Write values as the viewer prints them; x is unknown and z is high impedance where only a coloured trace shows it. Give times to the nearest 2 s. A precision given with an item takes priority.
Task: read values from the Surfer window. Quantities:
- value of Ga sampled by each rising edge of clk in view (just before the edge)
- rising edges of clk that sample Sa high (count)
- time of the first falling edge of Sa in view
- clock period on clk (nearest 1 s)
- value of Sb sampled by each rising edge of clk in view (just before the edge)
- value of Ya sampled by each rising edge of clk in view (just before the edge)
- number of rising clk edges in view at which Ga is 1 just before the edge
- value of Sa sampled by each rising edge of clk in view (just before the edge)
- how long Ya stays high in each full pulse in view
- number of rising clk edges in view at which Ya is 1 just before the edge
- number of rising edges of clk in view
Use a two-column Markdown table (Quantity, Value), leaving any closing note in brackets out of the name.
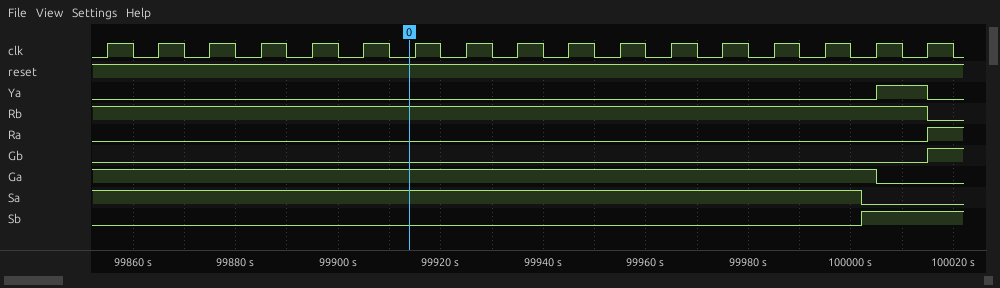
| Quantity | Value |
|---|---|
| value of Ga sampled by each rising edge of clk in view | 1 1 1 1 1 1 1 1 1 1 1 1 1 1 1 1 0 |
| rising edges of clk that sample Sa high | 15 |
| time of the first falling edge of Sa in view | 100002 s |
| clock period on clk | 10 s |
| value of Sb sampled by each rising edge of clk in view | 0 0 0 0 0 0 0 0 0 0 0 0 0 0 0 1 1 |
| value of Ya sampled by each rising edge of clk in view | 0 0 0 0 0 0 0 0 0 0 0 0 0 0 0 0 1 |
| number of rising clk edges in view at which Ga is 1 just before the edge | 16 |
| value of Sa sampled by each rising edge of clk in view | 1 1 1 1 1 1 1 1 1 1 1 1 1 1 1 0 0 |
| how long Ya stays high in each full pulse in view | 10 s |
| number of rising clk edges in view at which Ya is 1 just before the edge | 1 |
| number of rising edges of clk in view | 17 |
